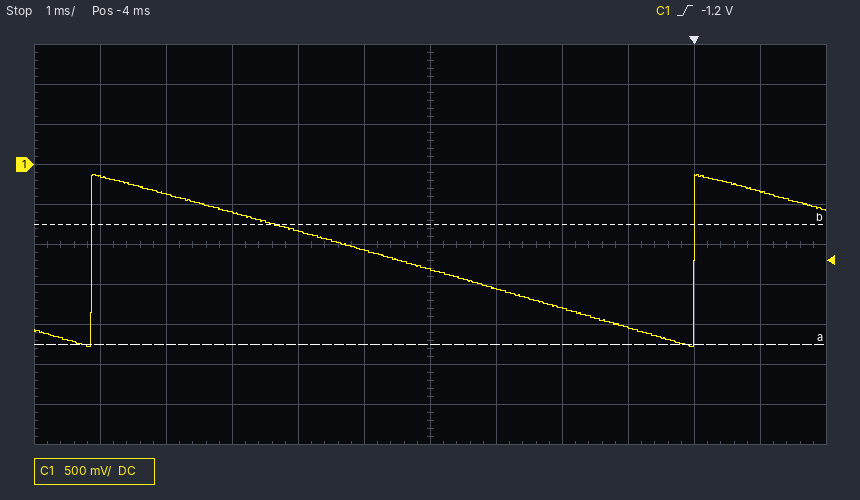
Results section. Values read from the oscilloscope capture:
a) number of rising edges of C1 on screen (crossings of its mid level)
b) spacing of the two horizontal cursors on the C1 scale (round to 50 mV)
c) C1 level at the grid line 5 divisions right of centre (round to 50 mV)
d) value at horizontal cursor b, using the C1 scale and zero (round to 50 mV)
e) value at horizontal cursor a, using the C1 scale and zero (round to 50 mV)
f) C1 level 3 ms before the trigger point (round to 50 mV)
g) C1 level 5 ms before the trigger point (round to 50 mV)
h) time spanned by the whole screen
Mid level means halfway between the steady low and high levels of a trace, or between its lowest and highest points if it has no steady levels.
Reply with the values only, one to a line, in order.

2
1.50 V
-350 mV
-750 mV
-2.25 V
-1.55 V
-1.05 V
12 ms
